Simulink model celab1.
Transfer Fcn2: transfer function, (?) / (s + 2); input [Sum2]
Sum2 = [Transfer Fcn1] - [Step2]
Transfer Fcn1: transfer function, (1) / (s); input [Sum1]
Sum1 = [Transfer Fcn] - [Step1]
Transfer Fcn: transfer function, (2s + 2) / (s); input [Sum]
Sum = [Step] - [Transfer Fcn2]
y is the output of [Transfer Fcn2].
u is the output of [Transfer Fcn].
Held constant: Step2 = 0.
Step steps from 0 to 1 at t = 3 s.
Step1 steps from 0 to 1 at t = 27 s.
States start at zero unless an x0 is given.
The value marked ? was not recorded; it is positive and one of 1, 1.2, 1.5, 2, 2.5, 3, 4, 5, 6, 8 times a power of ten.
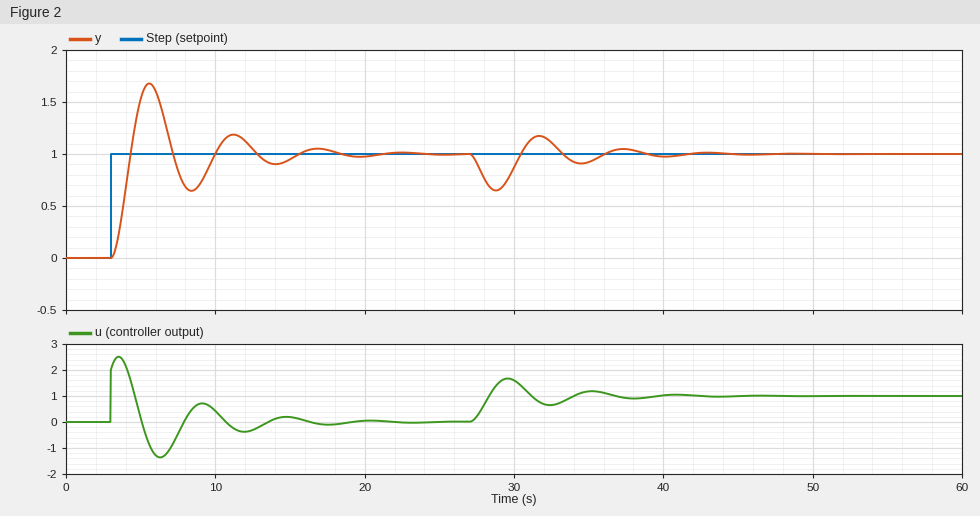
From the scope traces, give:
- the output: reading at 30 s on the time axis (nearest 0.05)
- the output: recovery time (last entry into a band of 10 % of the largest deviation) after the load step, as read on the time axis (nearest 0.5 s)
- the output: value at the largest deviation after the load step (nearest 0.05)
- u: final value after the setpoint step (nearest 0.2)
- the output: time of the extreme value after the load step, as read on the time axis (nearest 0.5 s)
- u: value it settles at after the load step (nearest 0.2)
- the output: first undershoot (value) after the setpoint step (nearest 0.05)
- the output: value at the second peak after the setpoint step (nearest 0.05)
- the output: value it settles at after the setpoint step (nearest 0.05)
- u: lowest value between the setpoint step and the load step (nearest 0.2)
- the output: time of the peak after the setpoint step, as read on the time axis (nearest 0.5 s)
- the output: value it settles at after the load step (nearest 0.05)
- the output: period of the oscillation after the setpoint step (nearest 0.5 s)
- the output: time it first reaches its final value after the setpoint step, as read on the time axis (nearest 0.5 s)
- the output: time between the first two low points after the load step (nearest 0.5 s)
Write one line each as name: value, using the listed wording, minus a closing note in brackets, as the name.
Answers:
the output: reading at 30 s on the time axis: 0.85
the output: recovery time (last entry into a band of 10 % of the largest deviation) after the load step, as read on the time axis: 38.0 s
the output: value at the largest deviation after the load step: 0.65
u: final value after the setpoint step: 0.0
the output: time of the extreme value after the load step, as read on the time axis: 29.0 s
u: value it settles at after the load step: 1.0
the output: first undershoot (value) after the setpoint step: 0.65
the output: value at the second peak after the setpoint step: 1.20
the output: value it settles at after the setpoint step: 1.00
u: lowest value between the setpoint step and the load step: -1.4
the output: time of the peak after the setpoint step, as read on the time axis: 5.5 s
the output: value it settles at after the load step: 1.00
the output: period of the oscillation after the setpoint step: 5.5 s
the output: time it first reaches its final value after the setpoint step, as read on the time axis: 4.5 s
the output: time between the first two low points after the load step: 5.5 s
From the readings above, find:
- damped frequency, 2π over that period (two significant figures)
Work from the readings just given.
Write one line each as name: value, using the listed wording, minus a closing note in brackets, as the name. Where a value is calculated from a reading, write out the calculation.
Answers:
damped frequency, 2π over that period: 2π / 5.5 = 1.1 rad/s
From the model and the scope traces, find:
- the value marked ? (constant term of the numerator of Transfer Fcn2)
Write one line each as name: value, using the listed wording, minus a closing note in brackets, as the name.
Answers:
the value marked ?: 1
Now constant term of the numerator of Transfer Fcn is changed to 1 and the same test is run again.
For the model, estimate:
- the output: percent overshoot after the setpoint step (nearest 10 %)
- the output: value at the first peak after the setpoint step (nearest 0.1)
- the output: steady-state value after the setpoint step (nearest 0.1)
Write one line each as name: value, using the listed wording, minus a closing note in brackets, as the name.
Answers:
the output: percent overshoot after the setpoint step: 40 %
the output: value at the first peak after the setpoint step: 1.4
the output: steady-state value after the setpoint step: 1.0
